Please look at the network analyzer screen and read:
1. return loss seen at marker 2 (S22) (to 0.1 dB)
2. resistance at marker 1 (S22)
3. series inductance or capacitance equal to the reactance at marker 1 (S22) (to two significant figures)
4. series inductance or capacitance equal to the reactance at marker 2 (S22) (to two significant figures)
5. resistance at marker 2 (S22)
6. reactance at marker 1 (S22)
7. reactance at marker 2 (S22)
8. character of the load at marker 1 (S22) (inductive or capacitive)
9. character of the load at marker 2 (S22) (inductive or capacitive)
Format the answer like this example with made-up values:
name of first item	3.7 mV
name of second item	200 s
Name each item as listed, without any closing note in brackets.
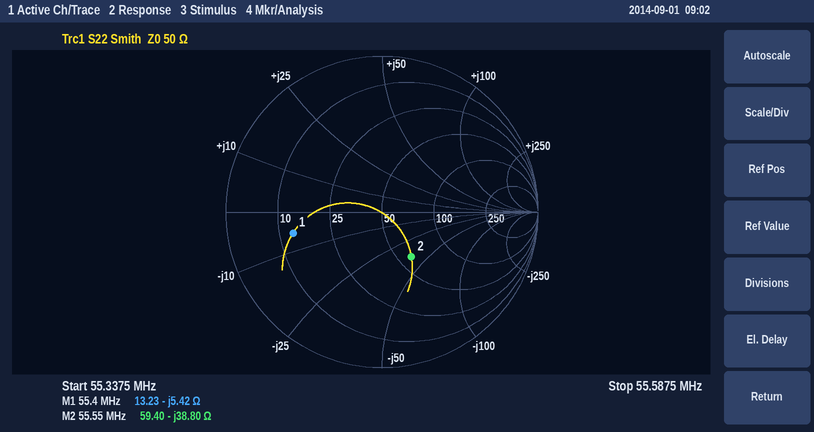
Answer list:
return loss seen at marker 2 (S22)	9.3 dB
resistance at marker 1	13.23 Ω
series inductance or capacitance equal to the reactance at marker 1 (S22)	530 pF
series inductance or capacitance equal to the reactance at marker 2 (S22)	74 pF
resistance at marker 2	59.40 Ω
reactance at marker 1	-5.42 Ω
reactance at marker 2	-38.80 Ω
character of the load at marker 1 (S22)	capacitive
character of the load at marker 2 (S22)	capacitive
